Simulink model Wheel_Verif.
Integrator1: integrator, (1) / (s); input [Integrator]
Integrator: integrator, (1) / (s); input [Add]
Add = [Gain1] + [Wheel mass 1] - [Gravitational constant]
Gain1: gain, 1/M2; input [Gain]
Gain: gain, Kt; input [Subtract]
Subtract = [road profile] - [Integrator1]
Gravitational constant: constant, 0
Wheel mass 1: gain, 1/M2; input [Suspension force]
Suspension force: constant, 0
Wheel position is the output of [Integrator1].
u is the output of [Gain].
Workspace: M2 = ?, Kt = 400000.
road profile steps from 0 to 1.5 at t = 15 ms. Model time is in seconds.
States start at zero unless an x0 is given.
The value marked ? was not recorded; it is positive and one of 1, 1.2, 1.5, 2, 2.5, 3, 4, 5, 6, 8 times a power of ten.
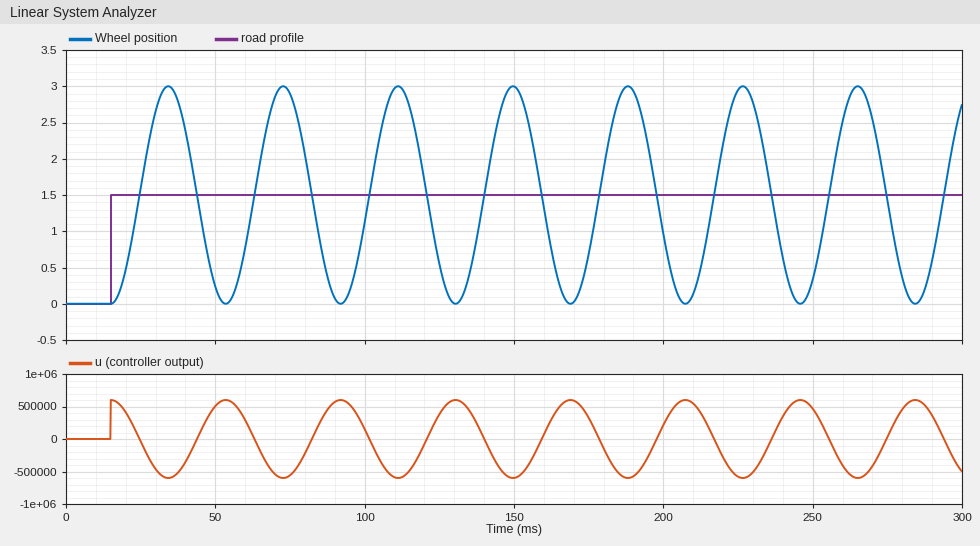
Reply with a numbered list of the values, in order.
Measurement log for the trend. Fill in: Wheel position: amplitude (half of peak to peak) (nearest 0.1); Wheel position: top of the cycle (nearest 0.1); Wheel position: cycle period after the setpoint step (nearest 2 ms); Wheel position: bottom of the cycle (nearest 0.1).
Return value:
1. 1.5
2. 3.0
3. 38 ms
4. 0.0
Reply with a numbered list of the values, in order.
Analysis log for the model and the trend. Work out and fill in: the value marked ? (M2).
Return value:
1. 15
